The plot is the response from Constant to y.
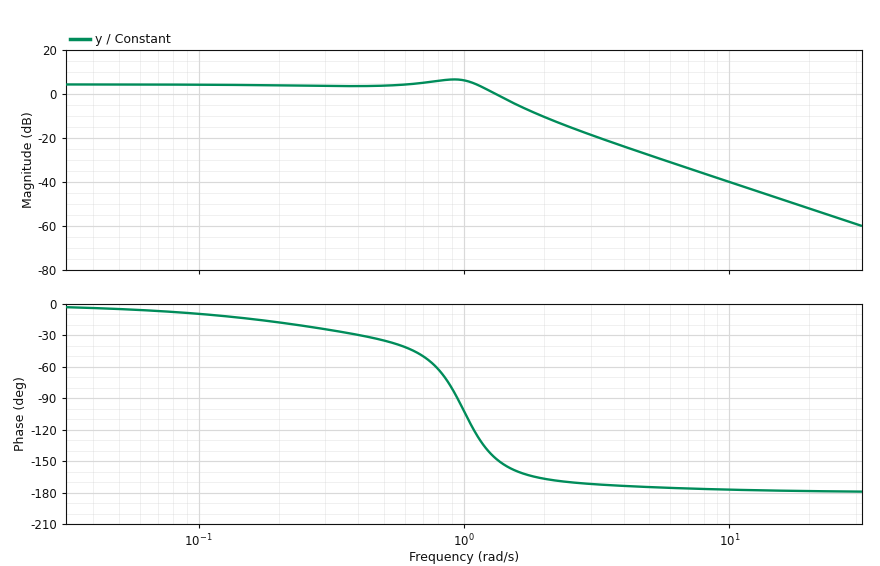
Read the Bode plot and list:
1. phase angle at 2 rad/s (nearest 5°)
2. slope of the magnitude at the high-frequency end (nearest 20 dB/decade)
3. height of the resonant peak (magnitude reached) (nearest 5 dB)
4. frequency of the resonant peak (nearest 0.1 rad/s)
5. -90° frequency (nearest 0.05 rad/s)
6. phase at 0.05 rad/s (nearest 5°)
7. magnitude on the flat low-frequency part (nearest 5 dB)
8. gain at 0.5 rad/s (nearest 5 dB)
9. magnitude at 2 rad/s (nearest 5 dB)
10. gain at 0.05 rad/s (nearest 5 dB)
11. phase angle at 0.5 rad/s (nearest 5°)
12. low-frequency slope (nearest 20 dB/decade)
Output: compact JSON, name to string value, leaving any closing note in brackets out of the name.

{"phase angle at 2 rad/s": "-165°", "slope of the magnitude at the high-frequency end": "-40 dB/decade", "height of the resonant peak (magnitude reached)": "5 dB", "frequency of the resonant peak": "0.9 rad/s", "-90° frequency": "0.95 rad/s", "phase at 0.05 rad/s": "-5°", "magnitude on the flat low-frequency part": "5 dB", "gain at 0.5 rad/s": "5 dB", "magnitude at 2 rad/s": "-10 dB", "gain at 0.05 rad/s": "5 dB", "phase angle at 0.5 rad/s": "-35°", "low-frequency slope": "0 dB/decade"}
